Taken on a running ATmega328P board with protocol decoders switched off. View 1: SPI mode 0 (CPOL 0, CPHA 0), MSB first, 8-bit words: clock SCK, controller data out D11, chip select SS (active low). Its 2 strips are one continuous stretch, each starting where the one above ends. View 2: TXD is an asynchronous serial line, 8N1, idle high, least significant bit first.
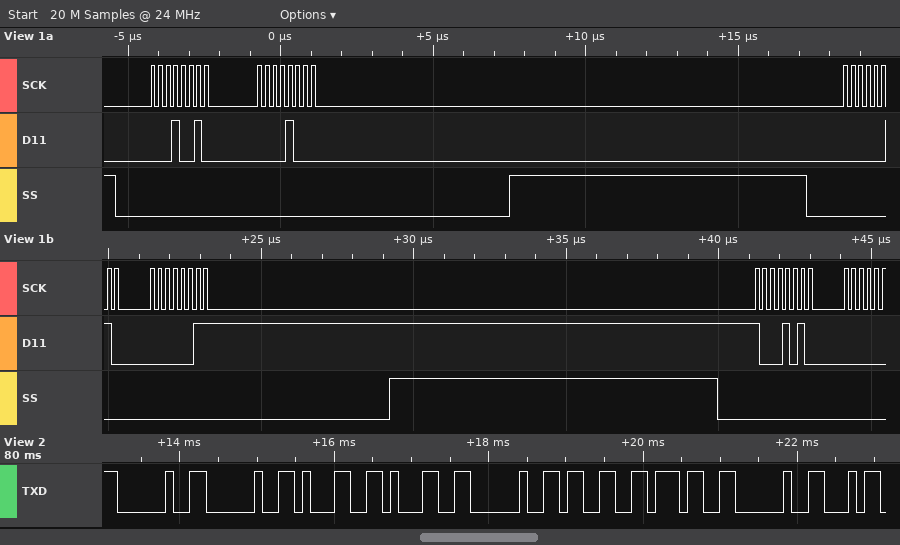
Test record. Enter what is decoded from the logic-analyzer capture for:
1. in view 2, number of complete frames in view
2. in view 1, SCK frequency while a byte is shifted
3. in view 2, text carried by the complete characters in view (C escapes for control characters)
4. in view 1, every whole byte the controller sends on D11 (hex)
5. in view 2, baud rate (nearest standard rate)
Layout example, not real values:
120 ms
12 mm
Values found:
8
4 MHz
"  11 37 "
12 08 02 03 8A
9600 baud
